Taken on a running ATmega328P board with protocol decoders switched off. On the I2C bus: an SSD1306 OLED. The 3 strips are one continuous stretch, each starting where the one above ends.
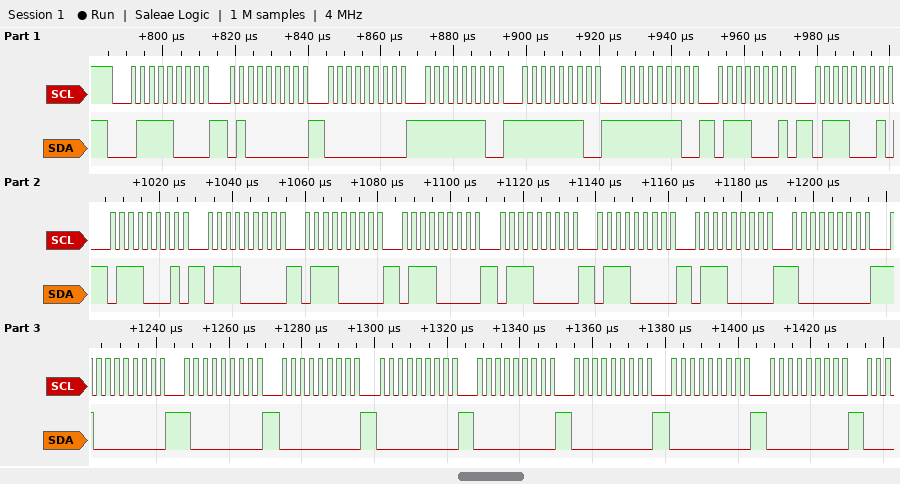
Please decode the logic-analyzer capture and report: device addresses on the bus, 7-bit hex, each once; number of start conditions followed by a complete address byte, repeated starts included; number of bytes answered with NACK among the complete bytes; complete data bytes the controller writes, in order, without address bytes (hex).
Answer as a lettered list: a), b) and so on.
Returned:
a) 0x3C
b) 1
c) 0
d) 40 00 FE FE FE 71 71 71 70 70 70 70 70 70 80 80 80 00 00 00 00 00 00
